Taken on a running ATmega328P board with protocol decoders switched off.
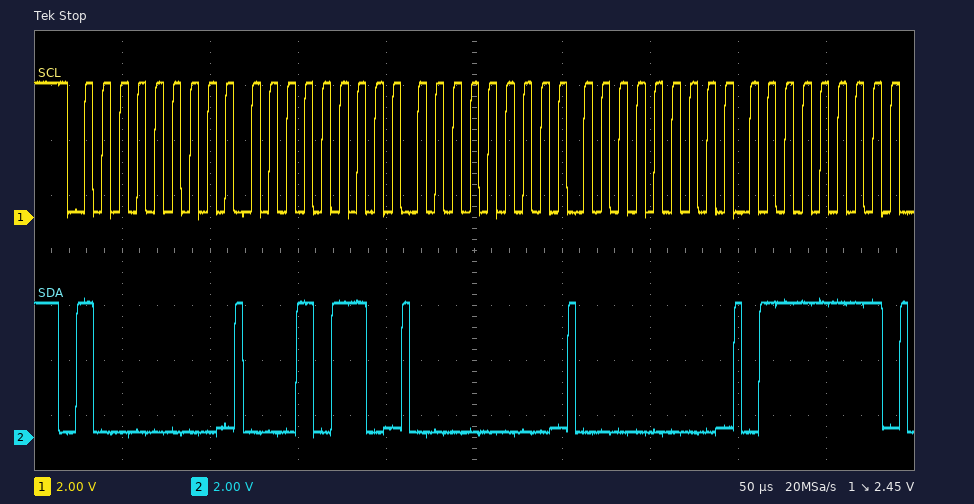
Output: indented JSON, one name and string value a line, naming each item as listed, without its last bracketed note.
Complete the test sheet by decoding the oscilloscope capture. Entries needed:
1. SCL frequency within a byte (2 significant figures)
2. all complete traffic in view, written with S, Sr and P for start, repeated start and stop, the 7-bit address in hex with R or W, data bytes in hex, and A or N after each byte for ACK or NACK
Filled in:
{
  "SCL frequency within a byte": "100 kHz",
  "all complete traffic in view, written with S, Sr and P for start, repeated start and stop, the 7-bit address in hex with R or W, data bytes in hex, and A or N after each byte for ACK or NACK": "S 40W A 16 A 00 A 00 A 7F A"
}
